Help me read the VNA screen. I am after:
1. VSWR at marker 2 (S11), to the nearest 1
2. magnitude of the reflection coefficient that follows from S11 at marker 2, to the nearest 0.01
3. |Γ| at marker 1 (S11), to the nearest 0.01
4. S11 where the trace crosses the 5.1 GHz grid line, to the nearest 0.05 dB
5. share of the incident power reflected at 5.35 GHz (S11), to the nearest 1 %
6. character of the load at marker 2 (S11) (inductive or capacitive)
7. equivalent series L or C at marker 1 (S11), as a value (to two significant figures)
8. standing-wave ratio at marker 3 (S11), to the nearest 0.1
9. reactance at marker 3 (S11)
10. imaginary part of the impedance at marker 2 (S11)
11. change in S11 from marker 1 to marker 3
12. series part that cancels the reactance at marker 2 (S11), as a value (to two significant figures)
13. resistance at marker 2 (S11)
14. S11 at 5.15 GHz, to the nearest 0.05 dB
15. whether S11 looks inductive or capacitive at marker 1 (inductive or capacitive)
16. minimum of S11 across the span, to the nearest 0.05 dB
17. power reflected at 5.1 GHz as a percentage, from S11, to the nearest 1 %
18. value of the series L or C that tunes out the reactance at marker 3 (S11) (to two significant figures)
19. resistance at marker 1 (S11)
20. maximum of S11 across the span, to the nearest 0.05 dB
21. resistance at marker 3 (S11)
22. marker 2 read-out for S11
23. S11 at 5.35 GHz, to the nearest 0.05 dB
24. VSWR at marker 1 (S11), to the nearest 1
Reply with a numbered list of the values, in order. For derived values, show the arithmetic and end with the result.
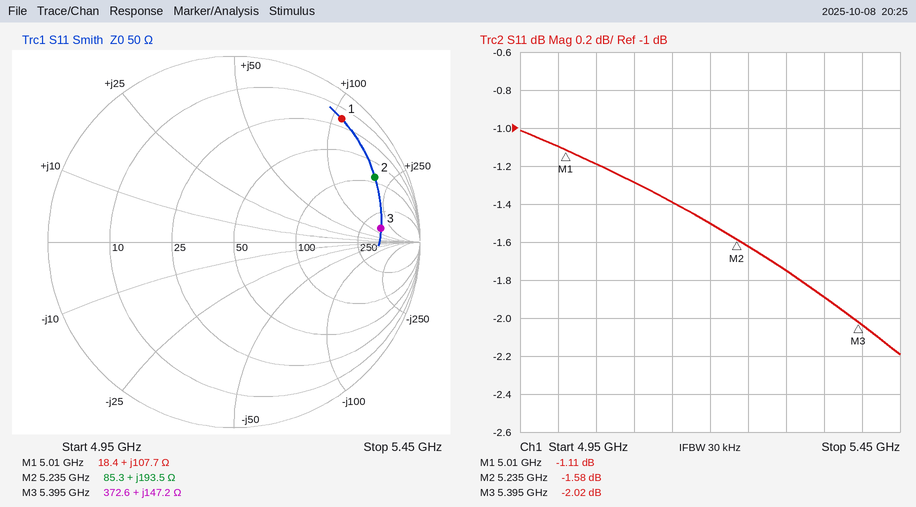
1. 11
2. 10^(-1.58/20) ≈ 0.83
3. 0.88
4. -1.30 dB
5. 10^(-1.9/10) ≈ 65 %
6. inductive
7. L = 107.7 Ω/(2π × 5.01 GHz) ≈ 3.4 nH
8. 8.6
9. +147.2 Ω
10. +193.5 Ω
11. -2.02 − (-1.11) = -0.91 dB
12. C = 1/(2π × 5.235 GHz × 193.5 Ω) ≈ 157 fF, so 160 fF to two significant figures
13. 85.3 Ω
14. -1.40 dB
15. inductive
16. -2.20 dB
17. 10^(-1.3/10) ≈ 74 %
18. C = 1/(2π × 5.395 GHz × 147.2 Ω) ≈ 200 fF
19. 18.4 Ω
20. -1.00 dB
21. 372.6 Ω
22. -1.58 dB
23. -1.90 dB
24. (1 + 0.8800)/(1 − 0.8800) ≈ 16
